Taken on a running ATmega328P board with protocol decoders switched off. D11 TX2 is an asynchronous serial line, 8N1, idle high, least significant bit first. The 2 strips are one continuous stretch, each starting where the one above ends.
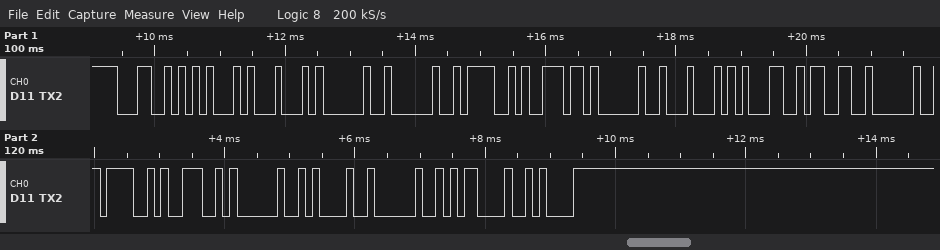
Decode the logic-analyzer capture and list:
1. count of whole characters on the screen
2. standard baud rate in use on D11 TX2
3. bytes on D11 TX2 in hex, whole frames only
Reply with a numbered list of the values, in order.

1. 19
2. 9600 baud
3. 4C 45 44 20 20 4F 6E 20 44 31 33 20 4F 4E 20 21 20 0D 0A
